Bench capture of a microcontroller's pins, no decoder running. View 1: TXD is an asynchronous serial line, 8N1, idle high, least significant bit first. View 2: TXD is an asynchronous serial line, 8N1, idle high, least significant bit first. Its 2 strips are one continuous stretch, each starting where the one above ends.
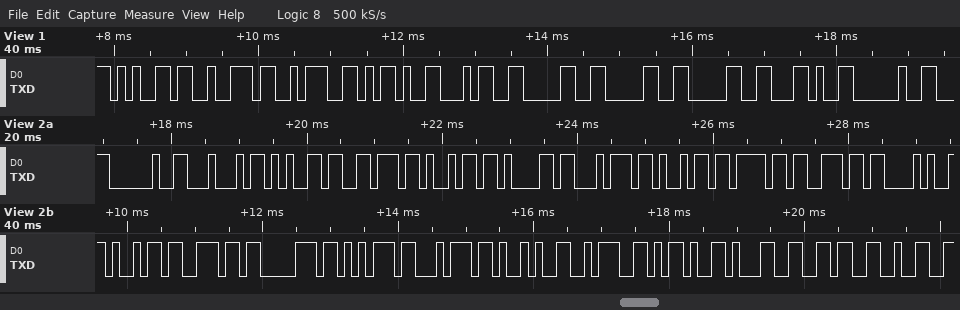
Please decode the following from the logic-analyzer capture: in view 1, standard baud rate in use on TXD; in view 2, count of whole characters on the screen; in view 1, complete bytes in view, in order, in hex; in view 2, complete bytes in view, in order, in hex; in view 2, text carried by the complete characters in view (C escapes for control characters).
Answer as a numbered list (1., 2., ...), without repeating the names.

1. 9600 baud
2. 22
3. 65 72 3A 2D 34 30 30 30 2C 20
4. 20 44 65 76 69 61 74 69 6F 6E 28 69 6E 70 75 74 29 3A 2D 31 36 32
5. " Deviation(input):-162"
